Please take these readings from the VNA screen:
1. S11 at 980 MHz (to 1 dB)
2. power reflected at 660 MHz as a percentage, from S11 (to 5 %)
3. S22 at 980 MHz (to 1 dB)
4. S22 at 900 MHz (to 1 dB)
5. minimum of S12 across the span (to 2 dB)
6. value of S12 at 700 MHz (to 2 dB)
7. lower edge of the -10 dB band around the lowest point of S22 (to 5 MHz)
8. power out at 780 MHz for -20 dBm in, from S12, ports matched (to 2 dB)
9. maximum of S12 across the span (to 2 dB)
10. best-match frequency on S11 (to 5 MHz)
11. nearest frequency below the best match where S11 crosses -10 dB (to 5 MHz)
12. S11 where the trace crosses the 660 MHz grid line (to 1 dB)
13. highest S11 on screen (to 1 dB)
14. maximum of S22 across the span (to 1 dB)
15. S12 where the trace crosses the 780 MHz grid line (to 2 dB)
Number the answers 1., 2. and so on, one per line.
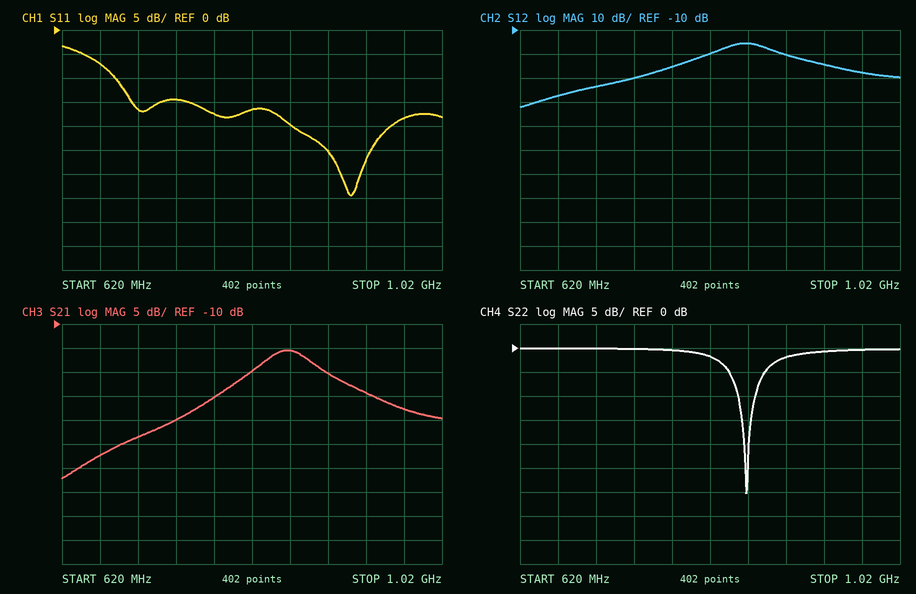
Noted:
1. -18 dB
2. 20 %
3. 0 dB
4. -2 dB
5. -42 dB
6. -34 dB
7. 850 MHz
8. -46 dBm
9. -16 dB
10. 925 MHz
11. 675 MHz
12. -7 dB
13. -3 dB
14. 0 dB
15. -26 dB
